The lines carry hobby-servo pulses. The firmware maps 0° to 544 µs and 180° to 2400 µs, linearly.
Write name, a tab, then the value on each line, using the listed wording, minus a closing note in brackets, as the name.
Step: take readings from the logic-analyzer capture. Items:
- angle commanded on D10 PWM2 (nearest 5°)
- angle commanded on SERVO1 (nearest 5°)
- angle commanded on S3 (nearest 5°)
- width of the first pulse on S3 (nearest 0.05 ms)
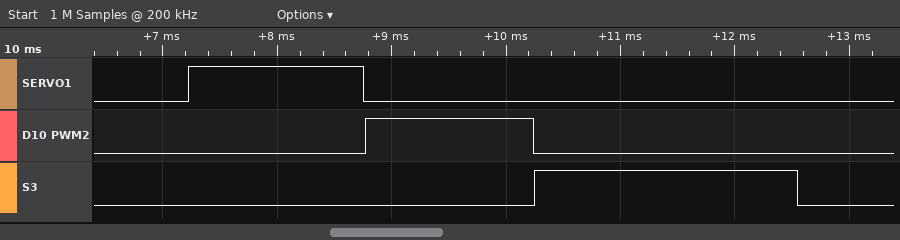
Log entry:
angle commanded on D10 PWM2	90°
angle commanded on SERVO1	95°
angle commanded on S3	170°
width of the first pulse on S3	2.30 ms
